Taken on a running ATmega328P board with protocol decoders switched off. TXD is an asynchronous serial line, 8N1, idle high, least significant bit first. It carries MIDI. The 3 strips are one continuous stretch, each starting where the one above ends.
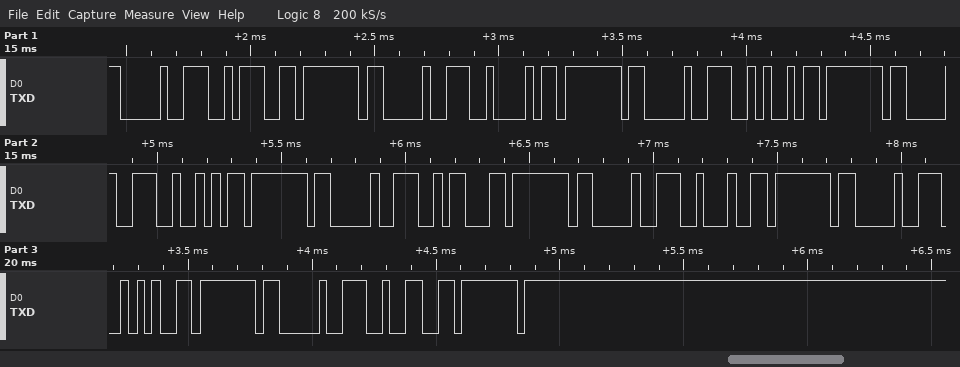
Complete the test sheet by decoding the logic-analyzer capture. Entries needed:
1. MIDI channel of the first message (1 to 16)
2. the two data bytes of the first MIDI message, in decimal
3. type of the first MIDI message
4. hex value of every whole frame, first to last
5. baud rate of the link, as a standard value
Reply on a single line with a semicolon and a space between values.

1; 58, 127; Note On; 90 3A 7F 90 42 7F 90 4A 7F 90 52 7F 90 1A 7F 90 22 7F 90 2A 7F 90 32 7F; 31250 baud
